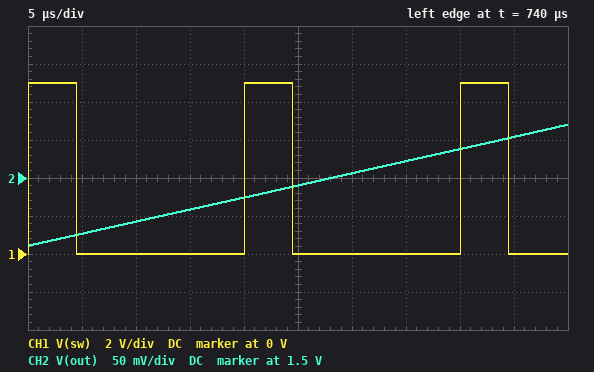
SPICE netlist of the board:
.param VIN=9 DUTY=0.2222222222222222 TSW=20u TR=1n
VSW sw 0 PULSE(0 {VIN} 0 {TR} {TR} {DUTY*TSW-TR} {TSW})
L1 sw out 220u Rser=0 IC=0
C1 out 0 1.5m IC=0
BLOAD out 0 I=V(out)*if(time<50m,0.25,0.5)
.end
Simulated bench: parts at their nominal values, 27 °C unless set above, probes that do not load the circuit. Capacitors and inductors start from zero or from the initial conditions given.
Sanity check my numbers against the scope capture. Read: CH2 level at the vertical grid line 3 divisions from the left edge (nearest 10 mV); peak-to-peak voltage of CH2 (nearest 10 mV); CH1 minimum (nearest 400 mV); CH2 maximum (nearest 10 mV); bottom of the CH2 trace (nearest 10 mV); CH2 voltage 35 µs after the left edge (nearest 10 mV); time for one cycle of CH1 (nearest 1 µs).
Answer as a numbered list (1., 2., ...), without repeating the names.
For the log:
1. 1.46 V
2. 160 mV
3. 0 V
4. 1.57 V
5. 1.41 V
6. 1.52 V
7. 20 µs
